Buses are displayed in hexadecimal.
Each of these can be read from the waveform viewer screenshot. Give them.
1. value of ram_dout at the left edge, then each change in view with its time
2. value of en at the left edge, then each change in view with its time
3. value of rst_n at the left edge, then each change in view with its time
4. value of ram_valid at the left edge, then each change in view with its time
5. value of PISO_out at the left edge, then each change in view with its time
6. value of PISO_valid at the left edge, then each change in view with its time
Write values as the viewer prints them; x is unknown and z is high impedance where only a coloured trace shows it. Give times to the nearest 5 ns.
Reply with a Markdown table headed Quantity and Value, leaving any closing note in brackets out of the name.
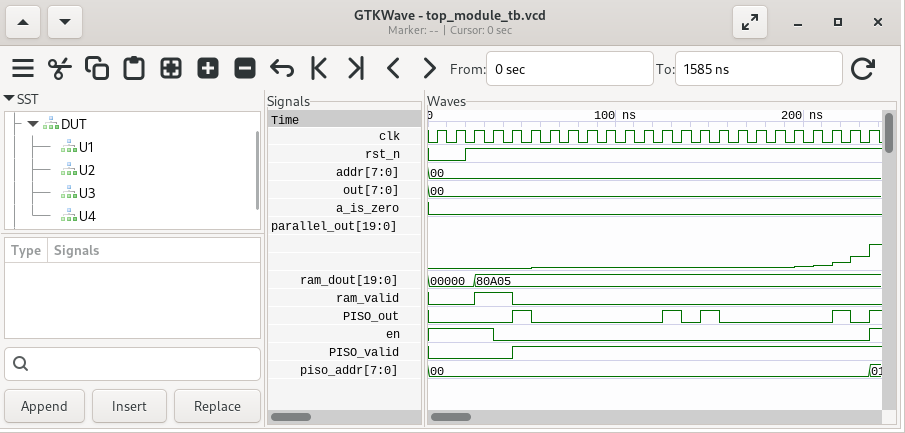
| Quantity | Value |
|---|---|
| value of ram_dout at the left edge, then each change in view with its time | 00000, 80A05 at 25 ns |
| value of en at the left edge, then each change in view with its time | 1, 0 at 35 ns, 1 at 235 ns |
| value of rst_n at the left edge, then each change in view with its time | 0, 1 at 20 ns |
| value of ram_valid at the left edge, then each change in view with its time | 0, 1 at 25 ns, 0 at 45 ns |
| value of PISO_out at the left edge, then each change in view with its time | 0, 1 at 45 ns, 0 at 55 ns, 1 at 125 ns, 0 at 135 ns, 1 at 145 ns, 0 at 155 ns, 1 at 215 ns, 0 at 225 ns, 1 at 235 ns |
| value of PISO_valid at the left edge, then each change in view with its time | 0, 1 at 45 ns |
